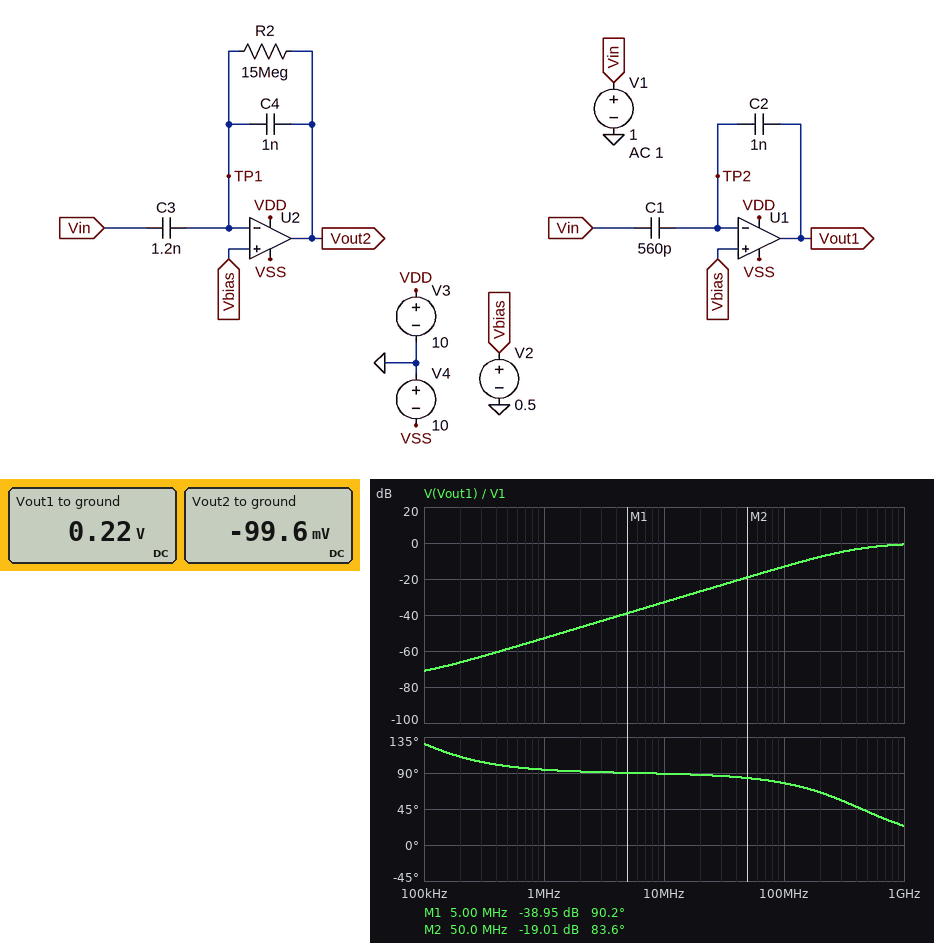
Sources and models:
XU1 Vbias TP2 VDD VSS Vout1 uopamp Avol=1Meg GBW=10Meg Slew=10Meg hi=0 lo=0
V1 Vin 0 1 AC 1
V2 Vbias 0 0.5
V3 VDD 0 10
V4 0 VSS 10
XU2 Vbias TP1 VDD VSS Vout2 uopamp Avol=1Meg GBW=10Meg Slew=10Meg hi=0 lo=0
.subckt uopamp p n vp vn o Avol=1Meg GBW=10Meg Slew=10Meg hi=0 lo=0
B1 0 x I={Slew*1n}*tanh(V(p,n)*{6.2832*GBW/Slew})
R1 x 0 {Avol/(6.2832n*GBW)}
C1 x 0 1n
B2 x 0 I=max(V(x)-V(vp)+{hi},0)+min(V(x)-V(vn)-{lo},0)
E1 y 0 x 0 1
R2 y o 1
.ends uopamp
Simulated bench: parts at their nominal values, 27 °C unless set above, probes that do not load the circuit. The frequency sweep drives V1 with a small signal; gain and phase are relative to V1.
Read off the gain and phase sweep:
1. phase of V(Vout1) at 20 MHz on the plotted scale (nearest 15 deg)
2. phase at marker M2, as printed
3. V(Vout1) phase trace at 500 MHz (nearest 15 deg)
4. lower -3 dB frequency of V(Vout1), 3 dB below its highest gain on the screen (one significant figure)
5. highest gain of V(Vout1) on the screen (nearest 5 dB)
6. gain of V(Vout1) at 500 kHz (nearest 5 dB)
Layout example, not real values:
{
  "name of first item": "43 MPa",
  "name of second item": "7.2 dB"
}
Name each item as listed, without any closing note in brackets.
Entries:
{
  "phase of V(Vout1) at 20 MHz on the plotted scale": "90 deg",
  "phase at marker M2, as printed": "83.6 deg",
  "V(Vout1) phase trace at 500 MHz": "45 deg",
  "lower -3 dB frequency of V(Vout1), 3 dB below its highest gain on the screen": "400 MHz",
  "highest gain of V(Vout1) on the screen": "0 dB",
  "gain of V(Vout1) at 500 kHz": "-60 dB"
}
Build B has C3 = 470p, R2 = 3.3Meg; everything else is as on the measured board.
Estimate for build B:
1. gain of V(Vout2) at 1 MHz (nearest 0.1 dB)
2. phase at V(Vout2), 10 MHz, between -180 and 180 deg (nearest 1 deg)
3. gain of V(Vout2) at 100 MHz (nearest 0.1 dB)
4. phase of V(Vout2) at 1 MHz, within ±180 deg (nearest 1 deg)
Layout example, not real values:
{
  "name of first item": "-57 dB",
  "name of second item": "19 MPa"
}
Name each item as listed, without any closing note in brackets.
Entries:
{
  "gain of V(Vout2) at 1 MHz": "-6.6 dB",
  "phase at V(Vout2), 10 MHz, between -180 and 180 deg": "123 deg",
  "gain of V(Vout2) at 100 MHz": "-12.7 dB",
  "phase of V(Vout2) at 1 MHz, within ±180 deg": "172 deg"
}
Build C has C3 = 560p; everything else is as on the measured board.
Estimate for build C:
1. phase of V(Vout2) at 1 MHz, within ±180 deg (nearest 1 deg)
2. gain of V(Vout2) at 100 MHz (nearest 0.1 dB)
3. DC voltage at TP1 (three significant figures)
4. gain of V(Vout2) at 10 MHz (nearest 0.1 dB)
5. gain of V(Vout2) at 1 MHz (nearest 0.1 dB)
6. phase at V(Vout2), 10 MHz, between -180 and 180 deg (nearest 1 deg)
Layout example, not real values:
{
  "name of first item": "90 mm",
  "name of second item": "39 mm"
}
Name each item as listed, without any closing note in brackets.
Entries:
{
  "phase of V(Vout2) at 1 MHz, within ±180 deg": "171 deg",
  "gain of V(Vout2) at 100 MHz": "-11.8 dB",
  "DC voltage at TP1": "500 mV",
  "gain of V(Vout2) at 10 MHz": "-9.8 dB",
  "gain of V(Vout2) at 1 MHz": "-5.1 dB",
  "phase at V(Vout2), 10 MHz, between -180 and 180 deg": "122 deg"
}
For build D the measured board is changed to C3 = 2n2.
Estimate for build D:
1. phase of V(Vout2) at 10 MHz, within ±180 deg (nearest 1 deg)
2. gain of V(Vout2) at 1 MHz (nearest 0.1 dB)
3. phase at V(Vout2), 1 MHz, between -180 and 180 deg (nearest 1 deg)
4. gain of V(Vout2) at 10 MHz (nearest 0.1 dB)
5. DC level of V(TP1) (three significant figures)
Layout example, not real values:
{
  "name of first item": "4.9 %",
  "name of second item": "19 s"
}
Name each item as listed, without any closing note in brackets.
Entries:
{
  "phase of V(Vout2) at 10 MHz, within ±180 deg": "105 deg",
  "gain of V(Vout2) at 1 MHz": "6.4 dB",
  "phase at V(Vout2), 1 MHz, between -180 and 180 deg": "162 deg",
  "gain of V(Vout2) at 10 MHz": "-3.0 dB",
  "DC level of V(TP1)": "500 mV"
}
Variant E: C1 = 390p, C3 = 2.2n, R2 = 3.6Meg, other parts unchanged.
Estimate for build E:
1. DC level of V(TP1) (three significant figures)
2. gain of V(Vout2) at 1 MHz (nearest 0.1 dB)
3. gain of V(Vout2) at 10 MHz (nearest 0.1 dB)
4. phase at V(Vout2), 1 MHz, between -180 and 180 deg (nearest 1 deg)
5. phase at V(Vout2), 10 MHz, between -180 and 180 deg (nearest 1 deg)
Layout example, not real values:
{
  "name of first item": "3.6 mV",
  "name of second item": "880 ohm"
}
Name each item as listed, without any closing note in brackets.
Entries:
{
  "DC level of V(TP1)": "500 mV",
  "gain of V(Vout2) at 1 MHz": "6.4 dB",
  "gain of V(Vout2) at 10 MHz": "-3.0 dB",
  "phase at V(Vout2), 1 MHz, between -180 and 180 deg": "162 deg",
  "phase at V(Vout2), 10 MHz, between -180 and 180 deg": "105 deg"
}
